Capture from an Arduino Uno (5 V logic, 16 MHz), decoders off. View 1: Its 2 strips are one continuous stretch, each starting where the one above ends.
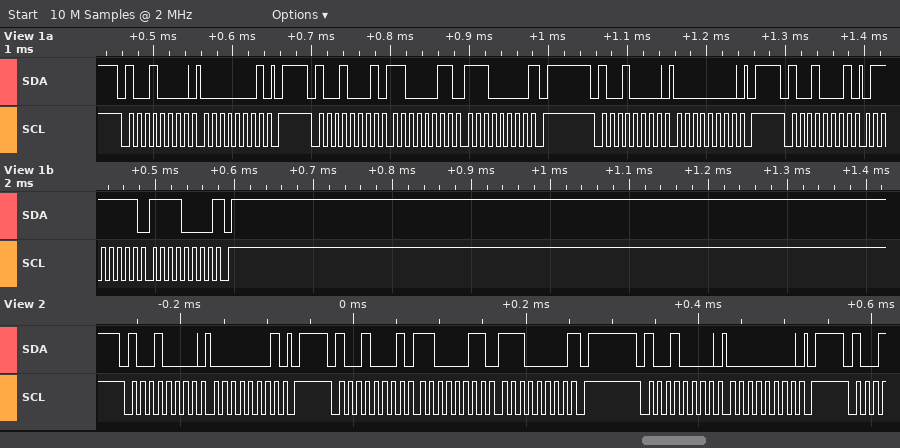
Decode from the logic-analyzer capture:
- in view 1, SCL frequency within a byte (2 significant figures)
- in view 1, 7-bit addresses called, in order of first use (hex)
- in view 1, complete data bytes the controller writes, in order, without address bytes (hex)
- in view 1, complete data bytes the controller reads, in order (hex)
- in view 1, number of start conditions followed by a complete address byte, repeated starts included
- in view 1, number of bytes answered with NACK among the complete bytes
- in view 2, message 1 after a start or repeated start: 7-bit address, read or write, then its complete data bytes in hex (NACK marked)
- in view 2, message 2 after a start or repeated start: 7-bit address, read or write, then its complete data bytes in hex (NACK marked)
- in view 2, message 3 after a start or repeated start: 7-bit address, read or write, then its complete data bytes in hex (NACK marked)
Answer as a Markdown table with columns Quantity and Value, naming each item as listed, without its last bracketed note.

| Quantity | Value |
|---|---|
| in view 1, SCL frequency within a byte | 100 kHz |
| in view 1, 7-bit addresses called, in order of first use | 0x48 |
| in view 1, complete data bytes the controller writes, in order, without address bytes | 01 00 |
| in view 1, complete data bytes the controller reads, in order | C3 E0 7F F0 |
| in view 1, number of start conditions followed by a complete address byte, repeated starts included | 4 |
| in view 1, number of bytes answered with NACK among the complete bytes | 2 |
| in view 2, message 1 after a start or repeated start: 7-bit address, read or write, then its complete data bytes in hex | 0x48 write: 01 |
| in view 2, message 2 after a start or repeated start: 7-bit address, read or write, then its complete data bytes in hex | 0x48 read: C3 E0 NACK |
| in view 2, message 3 after a start or repeated start: 7-bit address, read or write, then its complete data bytes in hex | 0x48 write: 00 |
